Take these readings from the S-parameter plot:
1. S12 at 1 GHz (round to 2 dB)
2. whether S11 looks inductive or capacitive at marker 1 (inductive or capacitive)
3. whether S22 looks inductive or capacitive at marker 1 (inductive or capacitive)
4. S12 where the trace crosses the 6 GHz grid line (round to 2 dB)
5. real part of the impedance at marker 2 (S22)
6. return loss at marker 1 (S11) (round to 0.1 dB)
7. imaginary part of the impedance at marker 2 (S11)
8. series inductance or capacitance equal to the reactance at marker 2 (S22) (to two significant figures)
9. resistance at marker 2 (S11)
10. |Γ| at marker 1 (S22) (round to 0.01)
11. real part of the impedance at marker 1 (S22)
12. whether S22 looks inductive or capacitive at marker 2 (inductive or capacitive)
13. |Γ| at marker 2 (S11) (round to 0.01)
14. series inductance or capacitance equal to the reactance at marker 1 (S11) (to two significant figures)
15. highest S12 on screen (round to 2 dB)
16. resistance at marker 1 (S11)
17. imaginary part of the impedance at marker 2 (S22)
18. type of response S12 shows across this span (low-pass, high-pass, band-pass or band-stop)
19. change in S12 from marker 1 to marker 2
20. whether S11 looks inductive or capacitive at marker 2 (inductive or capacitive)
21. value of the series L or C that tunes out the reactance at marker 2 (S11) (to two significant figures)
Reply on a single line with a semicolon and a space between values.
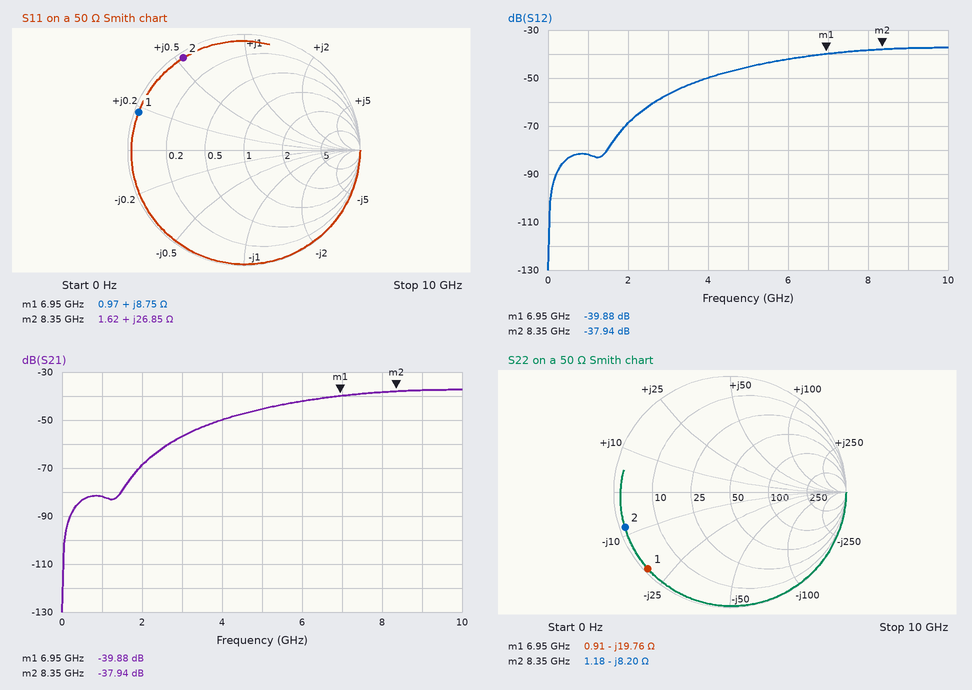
-82 dB; inductive; capacitive; -42 dB; 1.18 Ω; 0.3 dB; +26.85 Ω; 2.3 pF; 1.62 Ω; 0.97; 0.91 Ω; capacitive; 0.95; 200 pH; -38 dB; 0.97 Ω; -8.20 Ω; high-pass; 1.94 dB; inductive; 710 fF
